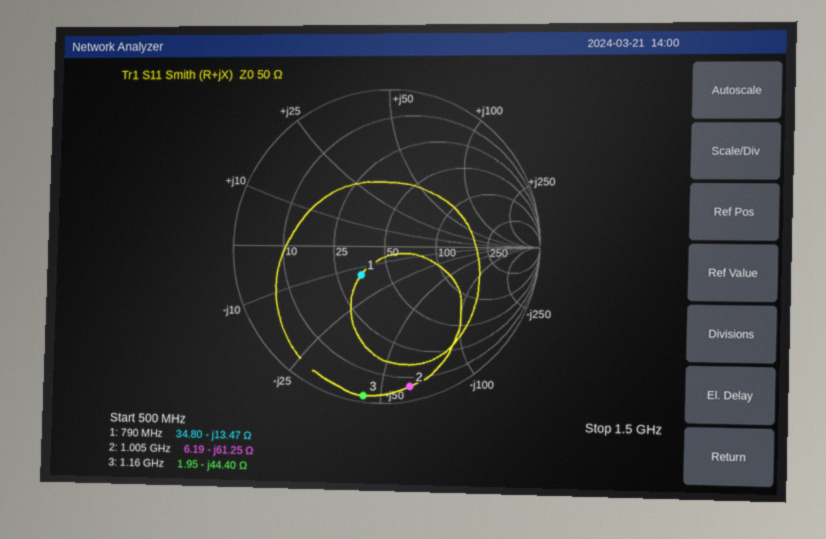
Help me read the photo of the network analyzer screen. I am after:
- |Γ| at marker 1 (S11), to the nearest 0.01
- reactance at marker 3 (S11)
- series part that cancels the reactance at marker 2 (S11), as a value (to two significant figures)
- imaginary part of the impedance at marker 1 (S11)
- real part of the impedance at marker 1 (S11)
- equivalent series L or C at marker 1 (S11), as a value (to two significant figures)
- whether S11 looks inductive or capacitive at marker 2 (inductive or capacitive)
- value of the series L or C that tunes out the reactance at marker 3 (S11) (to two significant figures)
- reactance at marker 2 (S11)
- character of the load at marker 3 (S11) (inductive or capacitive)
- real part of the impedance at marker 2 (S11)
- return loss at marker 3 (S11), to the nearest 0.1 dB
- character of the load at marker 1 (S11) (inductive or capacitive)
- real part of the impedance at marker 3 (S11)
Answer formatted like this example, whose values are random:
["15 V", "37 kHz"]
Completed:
["0.24", "-44.40 Ω", "9.7 nH", "-13.47 Ω", "34.80 Ω", "15 pF", "capacitive", "6.1 nH", "-61.25 Ω", "capacitive", "6.19 Ω", "0.4 dB", "capacitive", "1.95 Ω"]
